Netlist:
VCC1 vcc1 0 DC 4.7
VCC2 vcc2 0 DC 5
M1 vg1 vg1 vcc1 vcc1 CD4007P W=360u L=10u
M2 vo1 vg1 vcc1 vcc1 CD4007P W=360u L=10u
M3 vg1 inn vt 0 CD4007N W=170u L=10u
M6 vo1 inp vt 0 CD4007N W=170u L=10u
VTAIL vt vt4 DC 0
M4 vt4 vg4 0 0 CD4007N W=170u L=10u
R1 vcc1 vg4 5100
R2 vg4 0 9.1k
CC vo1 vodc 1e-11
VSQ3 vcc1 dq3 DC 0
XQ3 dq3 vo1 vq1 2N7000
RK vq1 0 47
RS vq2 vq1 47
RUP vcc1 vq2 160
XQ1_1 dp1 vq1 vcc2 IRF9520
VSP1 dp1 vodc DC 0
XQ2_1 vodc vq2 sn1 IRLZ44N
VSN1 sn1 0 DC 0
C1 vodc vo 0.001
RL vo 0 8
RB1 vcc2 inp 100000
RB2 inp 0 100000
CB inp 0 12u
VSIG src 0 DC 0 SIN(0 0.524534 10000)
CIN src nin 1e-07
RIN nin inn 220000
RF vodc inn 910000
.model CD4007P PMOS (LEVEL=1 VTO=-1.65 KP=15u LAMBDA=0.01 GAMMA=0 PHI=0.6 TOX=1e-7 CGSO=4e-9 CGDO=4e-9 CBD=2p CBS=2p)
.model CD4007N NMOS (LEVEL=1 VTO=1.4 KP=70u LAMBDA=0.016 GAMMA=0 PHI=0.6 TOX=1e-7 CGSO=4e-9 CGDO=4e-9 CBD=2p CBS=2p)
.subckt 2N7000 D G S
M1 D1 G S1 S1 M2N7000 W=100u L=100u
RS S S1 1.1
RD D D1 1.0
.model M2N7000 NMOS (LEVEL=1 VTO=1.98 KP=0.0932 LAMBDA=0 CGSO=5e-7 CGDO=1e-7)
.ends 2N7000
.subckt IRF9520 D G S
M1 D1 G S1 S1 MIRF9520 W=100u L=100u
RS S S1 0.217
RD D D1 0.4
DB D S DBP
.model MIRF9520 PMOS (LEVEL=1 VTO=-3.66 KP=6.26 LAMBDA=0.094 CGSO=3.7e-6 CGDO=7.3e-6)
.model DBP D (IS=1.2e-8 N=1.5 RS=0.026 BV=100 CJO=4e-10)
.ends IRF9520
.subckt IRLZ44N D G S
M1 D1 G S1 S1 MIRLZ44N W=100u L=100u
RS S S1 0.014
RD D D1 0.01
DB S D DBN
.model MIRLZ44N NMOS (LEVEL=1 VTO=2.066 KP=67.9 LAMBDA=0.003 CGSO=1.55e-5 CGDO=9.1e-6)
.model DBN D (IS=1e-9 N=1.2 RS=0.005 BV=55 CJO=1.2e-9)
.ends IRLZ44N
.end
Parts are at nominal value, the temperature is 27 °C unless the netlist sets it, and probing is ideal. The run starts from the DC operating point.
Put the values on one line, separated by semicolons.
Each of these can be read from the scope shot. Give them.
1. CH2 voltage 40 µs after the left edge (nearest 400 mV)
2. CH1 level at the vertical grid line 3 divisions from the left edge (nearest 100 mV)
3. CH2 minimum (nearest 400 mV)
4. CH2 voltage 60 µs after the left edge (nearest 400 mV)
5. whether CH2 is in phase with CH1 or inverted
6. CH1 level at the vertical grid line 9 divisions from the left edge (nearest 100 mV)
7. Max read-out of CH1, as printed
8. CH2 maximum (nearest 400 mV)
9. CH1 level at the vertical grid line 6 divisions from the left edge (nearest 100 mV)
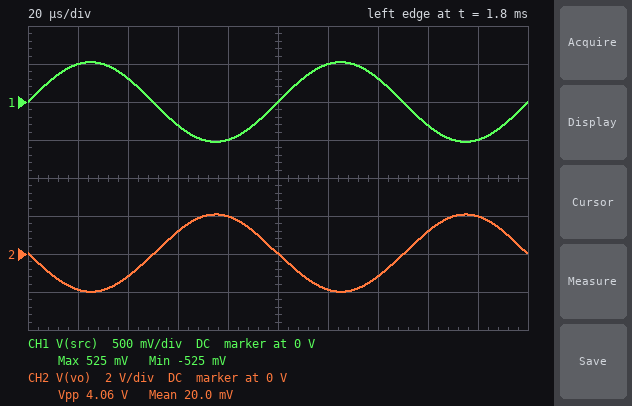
-1.2 V; -300 mV; -2.0 V; 1.2 V; inverted; -500 mV; 525 mV; 2.0 V; 500 mV
